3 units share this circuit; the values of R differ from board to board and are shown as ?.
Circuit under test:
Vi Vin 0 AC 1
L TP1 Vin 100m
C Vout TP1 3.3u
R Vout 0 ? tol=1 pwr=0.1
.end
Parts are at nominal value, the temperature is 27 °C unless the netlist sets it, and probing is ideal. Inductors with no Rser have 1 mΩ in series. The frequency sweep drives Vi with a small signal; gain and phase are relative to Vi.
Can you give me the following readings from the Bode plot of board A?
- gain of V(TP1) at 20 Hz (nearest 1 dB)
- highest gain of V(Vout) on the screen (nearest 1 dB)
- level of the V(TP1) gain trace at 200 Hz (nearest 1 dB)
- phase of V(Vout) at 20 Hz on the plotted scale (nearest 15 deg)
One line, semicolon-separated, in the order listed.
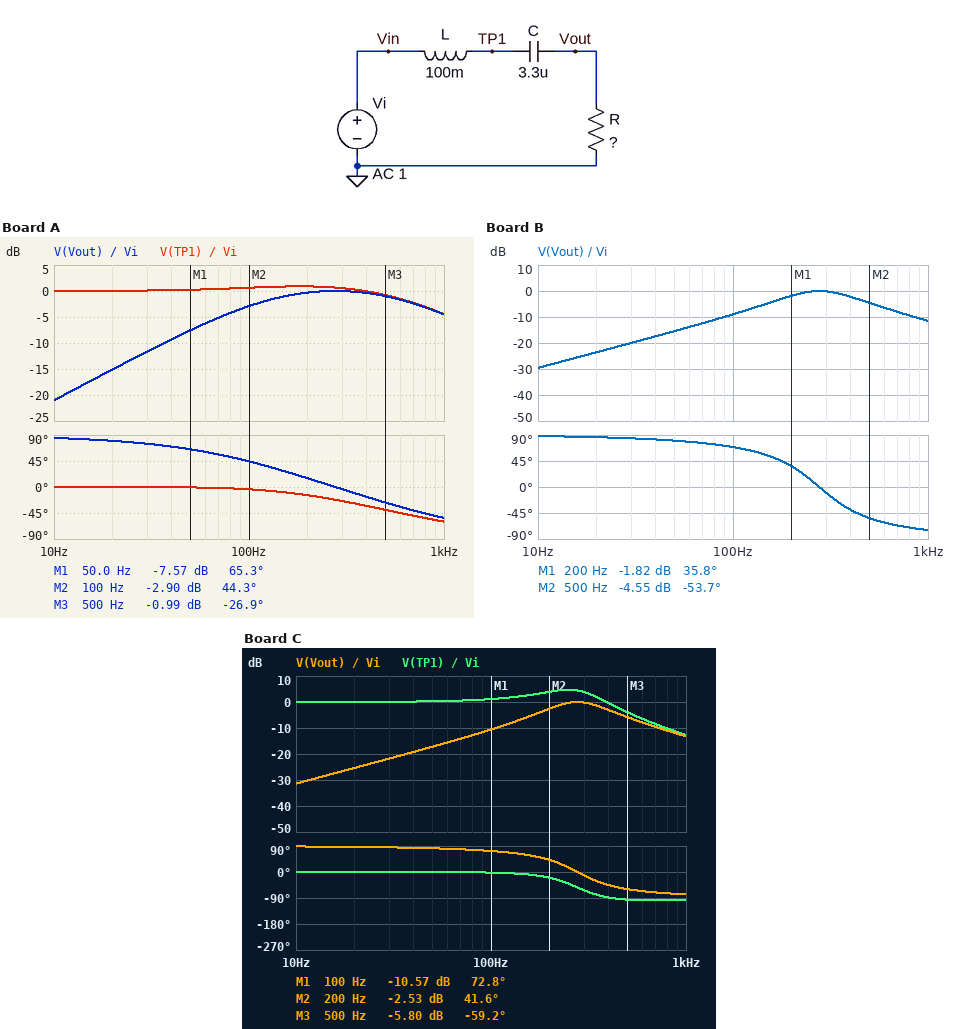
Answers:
0 dB; 0 dB; 1 dB; 75 deg
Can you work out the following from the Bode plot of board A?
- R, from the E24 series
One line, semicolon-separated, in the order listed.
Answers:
430 Ω
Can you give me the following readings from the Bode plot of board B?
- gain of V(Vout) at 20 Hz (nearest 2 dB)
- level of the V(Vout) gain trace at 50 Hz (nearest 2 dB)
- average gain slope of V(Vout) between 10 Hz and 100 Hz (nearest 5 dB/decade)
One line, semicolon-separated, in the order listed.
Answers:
-24 dB; -16 dB; 20 dB/decade
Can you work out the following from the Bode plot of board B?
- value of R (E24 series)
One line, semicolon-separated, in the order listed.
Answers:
160 Ω
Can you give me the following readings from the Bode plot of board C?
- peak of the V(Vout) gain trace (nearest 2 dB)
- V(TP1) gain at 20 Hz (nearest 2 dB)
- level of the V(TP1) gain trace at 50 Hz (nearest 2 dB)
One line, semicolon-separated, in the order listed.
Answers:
0 dB; 0 dB; 0 dB
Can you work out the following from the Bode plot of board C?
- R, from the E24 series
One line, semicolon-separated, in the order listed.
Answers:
130 Ω
